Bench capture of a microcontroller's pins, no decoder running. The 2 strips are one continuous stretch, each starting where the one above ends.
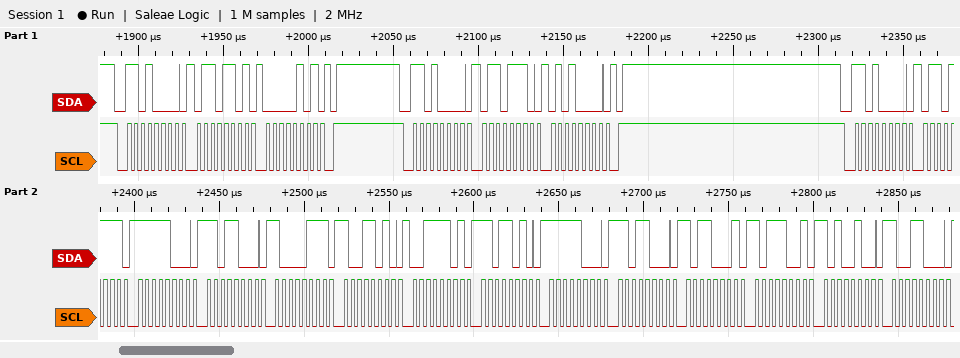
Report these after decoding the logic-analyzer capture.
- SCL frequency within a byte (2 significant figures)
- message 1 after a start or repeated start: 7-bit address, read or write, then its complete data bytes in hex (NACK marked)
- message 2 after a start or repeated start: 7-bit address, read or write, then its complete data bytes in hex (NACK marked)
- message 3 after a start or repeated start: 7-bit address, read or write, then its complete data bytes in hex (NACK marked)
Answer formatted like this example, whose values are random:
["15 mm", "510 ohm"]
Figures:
["250 kHz", "0x68 write: 6D 05", "0x68 write: 6E 50", "0x68 write: 6F F8 D8 87 9A 3D DA F8 D8 B1 B9 A4 98"]
